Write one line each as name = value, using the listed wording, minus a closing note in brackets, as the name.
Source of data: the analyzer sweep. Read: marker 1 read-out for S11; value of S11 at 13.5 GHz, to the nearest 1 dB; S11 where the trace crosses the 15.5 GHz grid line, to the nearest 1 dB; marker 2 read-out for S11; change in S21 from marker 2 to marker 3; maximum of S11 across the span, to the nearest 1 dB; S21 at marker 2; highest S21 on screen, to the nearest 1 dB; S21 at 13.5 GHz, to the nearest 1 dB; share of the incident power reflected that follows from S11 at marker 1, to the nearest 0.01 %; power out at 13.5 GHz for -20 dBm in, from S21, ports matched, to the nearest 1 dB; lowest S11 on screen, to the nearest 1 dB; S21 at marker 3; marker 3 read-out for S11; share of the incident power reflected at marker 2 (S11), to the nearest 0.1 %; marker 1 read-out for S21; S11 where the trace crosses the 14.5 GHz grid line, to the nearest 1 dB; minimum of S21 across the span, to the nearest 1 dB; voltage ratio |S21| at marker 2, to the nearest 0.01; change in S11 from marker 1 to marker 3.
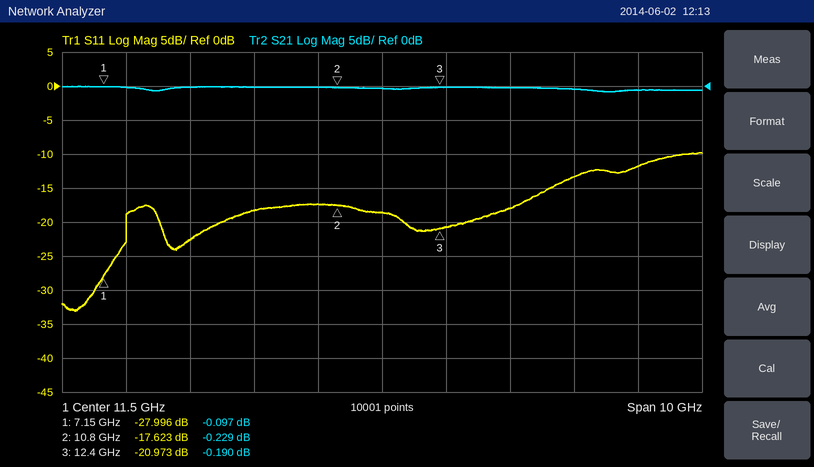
marker 1 read-out for S11 = -27.996 dB
value of S11 at 13.5 GHz, to the nearest 1 dB = -18 dB
S11 where the trace crosses the 15.5 GHz grid line, to the nearest 1 dB = -12 dB
marker 2 read-out for S11 = -17.623 dB
change in S21 from marker 2 to marker 3 = 0.039 dB
maximum of S11 across the span, to the nearest 1 dB = -10 dB
S21 at marker 2 = -0.229 dB
highest S21 on screen, to the nearest 1 dB = 0 dB
S21 at 13.5 GHz, to the nearest 1 dB = 0 dB
share of the incident power reflected that follows from S11 at marker 1, to the nearest 0.01 % = 0.16 %
power out at 13.5 GHz for -20 dBm in, from S21, ports matched, to the nearest 1 dB = -20 dBm
lowest S11 on screen, to the nearest 1 dB = -33 dB
S21 at marker 3 = -0.190 dB
marker 3 read-out for S11 = -20.973 dB
share of the incident power reflected at marker 2 (S11), to the nearest 0.1 % = 1.7 %
marker 1 read-out for S21 = -0.097 dB
S11 where the trace crosses the 14.5 GHz grid line, to the nearest 1 dB = -13 dB
minimum of S21 across the span, to the nearest 1 dB = -1 dB
voltage ratio |S21| at marker 2, to the nearest 0.01 = 0.97
change in S11 from marker 1 to marker 3 = 7.023 dB
